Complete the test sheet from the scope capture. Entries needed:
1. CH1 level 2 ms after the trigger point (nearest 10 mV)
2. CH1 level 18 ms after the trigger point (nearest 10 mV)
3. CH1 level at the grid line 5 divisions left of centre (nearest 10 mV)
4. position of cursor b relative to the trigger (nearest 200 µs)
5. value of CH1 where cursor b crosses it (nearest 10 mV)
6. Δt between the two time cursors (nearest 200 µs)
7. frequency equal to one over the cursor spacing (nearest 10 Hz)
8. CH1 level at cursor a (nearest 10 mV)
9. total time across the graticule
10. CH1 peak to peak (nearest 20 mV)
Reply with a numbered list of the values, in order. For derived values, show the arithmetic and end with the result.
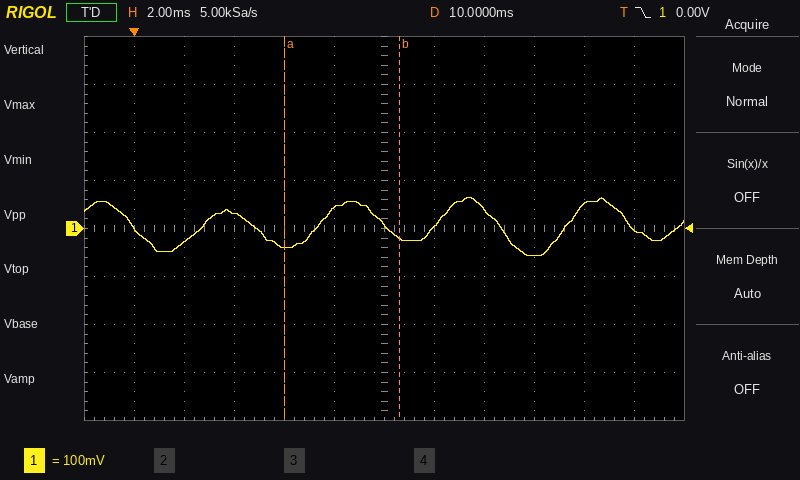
1. -30 mV
2. 50 mV
3. 0 mV
4. +10.6 ms
5. -20 mV
6. 4.6 ms
7. 1 / 4.6 ms ≈ 220 Hz
8. -40 mV
9. 24 ms
10. 120 mV
